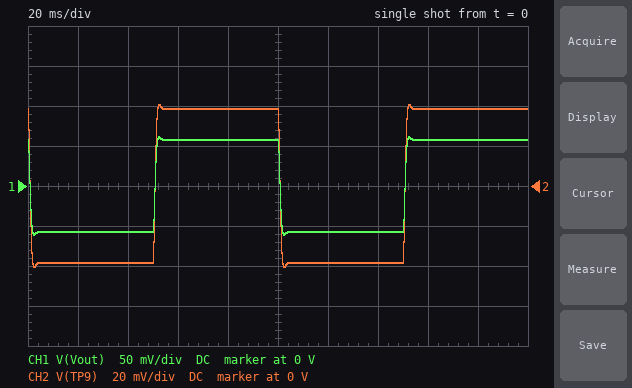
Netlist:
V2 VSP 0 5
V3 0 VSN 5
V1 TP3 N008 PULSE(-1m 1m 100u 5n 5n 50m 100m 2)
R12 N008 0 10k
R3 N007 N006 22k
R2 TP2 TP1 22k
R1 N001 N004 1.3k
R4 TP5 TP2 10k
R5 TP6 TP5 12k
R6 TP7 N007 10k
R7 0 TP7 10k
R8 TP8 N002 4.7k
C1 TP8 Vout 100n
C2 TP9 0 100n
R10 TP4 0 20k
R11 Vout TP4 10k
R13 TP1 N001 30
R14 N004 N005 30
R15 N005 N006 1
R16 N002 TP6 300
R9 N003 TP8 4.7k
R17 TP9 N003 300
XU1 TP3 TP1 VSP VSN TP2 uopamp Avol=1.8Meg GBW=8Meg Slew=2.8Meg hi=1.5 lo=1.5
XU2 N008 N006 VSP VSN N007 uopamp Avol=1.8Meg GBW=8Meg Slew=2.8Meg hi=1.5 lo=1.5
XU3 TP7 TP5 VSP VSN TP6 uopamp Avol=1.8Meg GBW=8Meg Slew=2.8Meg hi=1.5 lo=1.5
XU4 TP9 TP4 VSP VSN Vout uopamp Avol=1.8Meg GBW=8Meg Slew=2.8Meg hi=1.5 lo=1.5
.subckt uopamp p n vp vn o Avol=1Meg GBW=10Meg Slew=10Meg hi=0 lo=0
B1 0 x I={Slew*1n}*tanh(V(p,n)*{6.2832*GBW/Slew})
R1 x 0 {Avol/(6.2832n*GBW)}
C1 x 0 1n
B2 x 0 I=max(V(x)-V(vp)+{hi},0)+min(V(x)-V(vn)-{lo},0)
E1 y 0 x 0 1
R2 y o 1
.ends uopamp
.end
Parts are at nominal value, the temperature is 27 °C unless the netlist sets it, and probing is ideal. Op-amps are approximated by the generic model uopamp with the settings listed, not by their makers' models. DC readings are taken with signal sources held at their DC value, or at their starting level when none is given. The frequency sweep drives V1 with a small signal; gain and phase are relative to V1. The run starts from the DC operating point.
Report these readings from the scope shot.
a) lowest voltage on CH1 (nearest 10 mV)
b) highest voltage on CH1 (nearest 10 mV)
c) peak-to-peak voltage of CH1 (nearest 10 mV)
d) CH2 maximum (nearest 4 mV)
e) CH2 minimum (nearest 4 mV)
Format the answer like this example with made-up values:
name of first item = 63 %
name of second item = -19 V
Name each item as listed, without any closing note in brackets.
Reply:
lowest voltage on CH1 = -60 mV
highest voltage on CH1 = 60 mV
peak-to-peak voltage of CH1 = 120 mV
CH2 maximum = 40 mV
CH2 minimum = -40 mV
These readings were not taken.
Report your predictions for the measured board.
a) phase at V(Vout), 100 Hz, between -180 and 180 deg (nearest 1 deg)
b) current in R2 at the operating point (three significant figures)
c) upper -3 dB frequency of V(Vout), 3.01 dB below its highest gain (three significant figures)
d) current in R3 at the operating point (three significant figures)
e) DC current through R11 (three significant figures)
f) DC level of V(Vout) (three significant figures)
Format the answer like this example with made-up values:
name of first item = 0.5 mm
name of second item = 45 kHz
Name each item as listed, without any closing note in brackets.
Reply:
phase at V(Vout), 100 Hz, between -180 and 180 deg = 152 deg
current in R2 at the operating point = 735 nA
upper -3 dB frequency of V(Vout), 3.01 dB below its highest gain = 299 Hz
current in R3 at the operating point = 735 nA
DC current through R11 = 1.92 µA
DC level of V(Vout) = 57.6 mV
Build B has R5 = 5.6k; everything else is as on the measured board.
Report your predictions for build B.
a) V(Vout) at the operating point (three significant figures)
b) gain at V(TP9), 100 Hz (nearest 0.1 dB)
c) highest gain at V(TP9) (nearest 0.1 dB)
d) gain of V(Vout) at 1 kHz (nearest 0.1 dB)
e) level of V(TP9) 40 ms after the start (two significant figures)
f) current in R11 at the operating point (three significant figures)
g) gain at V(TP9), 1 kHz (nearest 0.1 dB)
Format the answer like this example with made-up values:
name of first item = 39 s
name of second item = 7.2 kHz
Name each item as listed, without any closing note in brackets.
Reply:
V(Vout) at the operating point = 33.3 mV
gain at V(TP9), 100 Hz = 26.8 dB
highest gain at V(TP9) = 26.9 dB
gain of V(Vout) at 1 kHz = 10.4 dB
level of V(TP9) 40 ms after the start = -22 mV
current in R11 at the operating point = 1.11 µA
gain at V(TP9), 1 kHz = 6.9 dB
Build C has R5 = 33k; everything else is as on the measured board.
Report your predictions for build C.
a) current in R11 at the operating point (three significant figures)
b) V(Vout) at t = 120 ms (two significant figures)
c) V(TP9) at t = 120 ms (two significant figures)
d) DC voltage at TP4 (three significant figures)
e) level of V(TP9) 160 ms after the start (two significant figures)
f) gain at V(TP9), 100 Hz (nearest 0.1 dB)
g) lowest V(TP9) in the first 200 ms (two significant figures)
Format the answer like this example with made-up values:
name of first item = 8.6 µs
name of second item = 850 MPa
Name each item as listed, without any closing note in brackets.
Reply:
current in R11 at the operating point = 4.57 µA
V(Vout) at t = 120 ms = -140 mV
V(TP9) at t = 120 ms = -91 mV
DC voltage at TP4 = 91.4 mV
level of V(TP9) 160 ms after the start = 91 mV
gain at V(TP9), 100 Hz = 39.1 dB
lowest V(TP9) in the first 200 ms = -97 mV
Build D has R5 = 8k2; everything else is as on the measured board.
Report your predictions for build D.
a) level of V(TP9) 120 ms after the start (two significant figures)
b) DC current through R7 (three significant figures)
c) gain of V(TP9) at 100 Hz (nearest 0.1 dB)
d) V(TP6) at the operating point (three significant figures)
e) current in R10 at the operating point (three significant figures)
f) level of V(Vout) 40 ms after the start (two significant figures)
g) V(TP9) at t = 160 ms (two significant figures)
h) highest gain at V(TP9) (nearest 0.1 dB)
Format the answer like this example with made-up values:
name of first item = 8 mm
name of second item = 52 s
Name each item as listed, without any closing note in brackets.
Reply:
level of V(TP9) 120 ms after the start = -29 mV
DC current through R7 = 808 nA
gain of V(TP9) at 100 Hz = 29.0 dB
V(TP6) at the operating point = 28.8 mV
current in R10 at the operating point = 1.44 µA
level of V(Vout) 40 ms after the start = -43 mV
V(TP9) at t = 160 ms = 29 mV
highest gain at V(TP9) = 29.2 dB
